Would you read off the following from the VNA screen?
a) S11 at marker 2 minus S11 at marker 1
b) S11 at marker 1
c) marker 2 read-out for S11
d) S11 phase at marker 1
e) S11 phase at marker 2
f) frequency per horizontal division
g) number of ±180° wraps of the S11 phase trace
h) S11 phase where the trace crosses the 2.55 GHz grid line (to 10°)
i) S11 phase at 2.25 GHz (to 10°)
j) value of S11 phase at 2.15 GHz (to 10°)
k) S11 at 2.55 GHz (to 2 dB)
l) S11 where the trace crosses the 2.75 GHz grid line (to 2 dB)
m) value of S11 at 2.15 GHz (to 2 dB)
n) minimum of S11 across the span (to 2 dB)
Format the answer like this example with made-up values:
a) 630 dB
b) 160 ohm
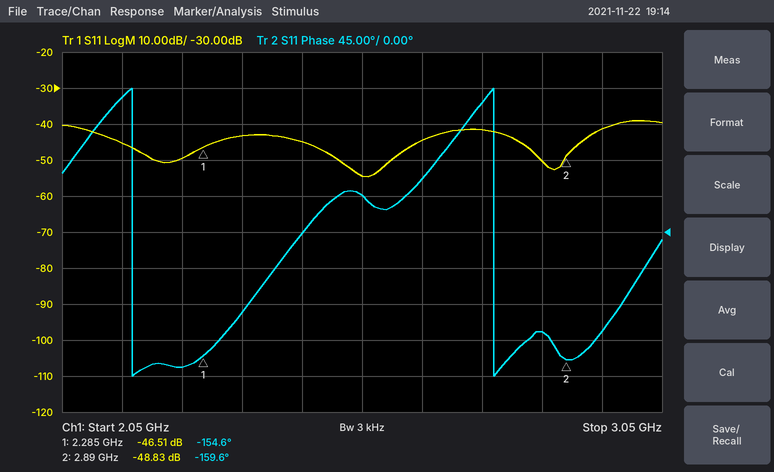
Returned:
a) -2.32 dB
b) -46.51 dB
c) -48.83 dB
d) -154.6°
e) -159.6°
f) 100 MHz
g) 2
h) 50°
i) -170°
j) 170°
k) -54 dB
l) -42 dB
m) -46 dB
n) -54 dB
